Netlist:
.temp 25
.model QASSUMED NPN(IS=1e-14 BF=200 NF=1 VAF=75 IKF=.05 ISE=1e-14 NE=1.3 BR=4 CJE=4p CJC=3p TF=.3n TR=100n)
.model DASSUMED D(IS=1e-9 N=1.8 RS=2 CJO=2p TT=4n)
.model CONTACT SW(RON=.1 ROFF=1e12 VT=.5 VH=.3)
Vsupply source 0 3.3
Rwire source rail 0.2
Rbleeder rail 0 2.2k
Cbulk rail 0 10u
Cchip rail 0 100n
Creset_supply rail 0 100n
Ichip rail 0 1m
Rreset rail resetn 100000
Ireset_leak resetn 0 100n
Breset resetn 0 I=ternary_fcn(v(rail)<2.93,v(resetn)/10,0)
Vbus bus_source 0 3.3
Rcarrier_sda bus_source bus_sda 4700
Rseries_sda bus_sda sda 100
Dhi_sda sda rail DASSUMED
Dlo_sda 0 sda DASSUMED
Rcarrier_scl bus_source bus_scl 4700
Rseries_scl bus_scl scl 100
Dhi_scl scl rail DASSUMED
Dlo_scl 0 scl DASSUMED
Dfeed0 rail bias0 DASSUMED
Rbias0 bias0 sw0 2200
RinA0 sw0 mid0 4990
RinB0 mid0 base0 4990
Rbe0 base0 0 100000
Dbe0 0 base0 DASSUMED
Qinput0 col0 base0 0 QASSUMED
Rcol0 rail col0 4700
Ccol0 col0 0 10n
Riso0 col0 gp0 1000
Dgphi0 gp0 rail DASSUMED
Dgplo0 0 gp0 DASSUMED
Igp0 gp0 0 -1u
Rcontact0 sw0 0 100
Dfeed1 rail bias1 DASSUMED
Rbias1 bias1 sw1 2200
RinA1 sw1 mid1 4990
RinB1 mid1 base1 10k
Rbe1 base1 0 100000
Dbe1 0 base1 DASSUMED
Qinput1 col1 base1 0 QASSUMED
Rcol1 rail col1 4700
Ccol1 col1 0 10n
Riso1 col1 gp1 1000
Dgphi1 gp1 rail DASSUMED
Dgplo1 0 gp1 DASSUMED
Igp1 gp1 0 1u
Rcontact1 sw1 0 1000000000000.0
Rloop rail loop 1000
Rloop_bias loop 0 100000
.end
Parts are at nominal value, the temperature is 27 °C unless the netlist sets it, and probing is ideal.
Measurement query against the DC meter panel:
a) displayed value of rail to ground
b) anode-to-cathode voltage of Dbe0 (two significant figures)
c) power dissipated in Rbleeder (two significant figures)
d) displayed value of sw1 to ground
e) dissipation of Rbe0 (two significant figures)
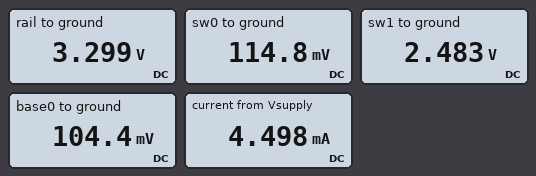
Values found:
3.299 V
-100 mV
4.9 mW
2.483 V
110 nW
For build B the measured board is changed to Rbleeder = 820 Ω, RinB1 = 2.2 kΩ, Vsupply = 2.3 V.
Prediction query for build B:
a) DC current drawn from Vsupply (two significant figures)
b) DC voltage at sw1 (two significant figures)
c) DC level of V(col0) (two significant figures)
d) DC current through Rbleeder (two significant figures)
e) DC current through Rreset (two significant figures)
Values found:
5.0 mA
1.5 V
2.3 V
2.8 mA
23 µA
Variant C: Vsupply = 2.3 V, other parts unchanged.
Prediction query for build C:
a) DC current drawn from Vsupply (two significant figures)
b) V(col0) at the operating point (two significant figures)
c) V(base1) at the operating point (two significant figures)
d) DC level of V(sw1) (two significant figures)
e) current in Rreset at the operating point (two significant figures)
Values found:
3.2 mA
2.3 V
650 mV
1.6 V
23 µA
